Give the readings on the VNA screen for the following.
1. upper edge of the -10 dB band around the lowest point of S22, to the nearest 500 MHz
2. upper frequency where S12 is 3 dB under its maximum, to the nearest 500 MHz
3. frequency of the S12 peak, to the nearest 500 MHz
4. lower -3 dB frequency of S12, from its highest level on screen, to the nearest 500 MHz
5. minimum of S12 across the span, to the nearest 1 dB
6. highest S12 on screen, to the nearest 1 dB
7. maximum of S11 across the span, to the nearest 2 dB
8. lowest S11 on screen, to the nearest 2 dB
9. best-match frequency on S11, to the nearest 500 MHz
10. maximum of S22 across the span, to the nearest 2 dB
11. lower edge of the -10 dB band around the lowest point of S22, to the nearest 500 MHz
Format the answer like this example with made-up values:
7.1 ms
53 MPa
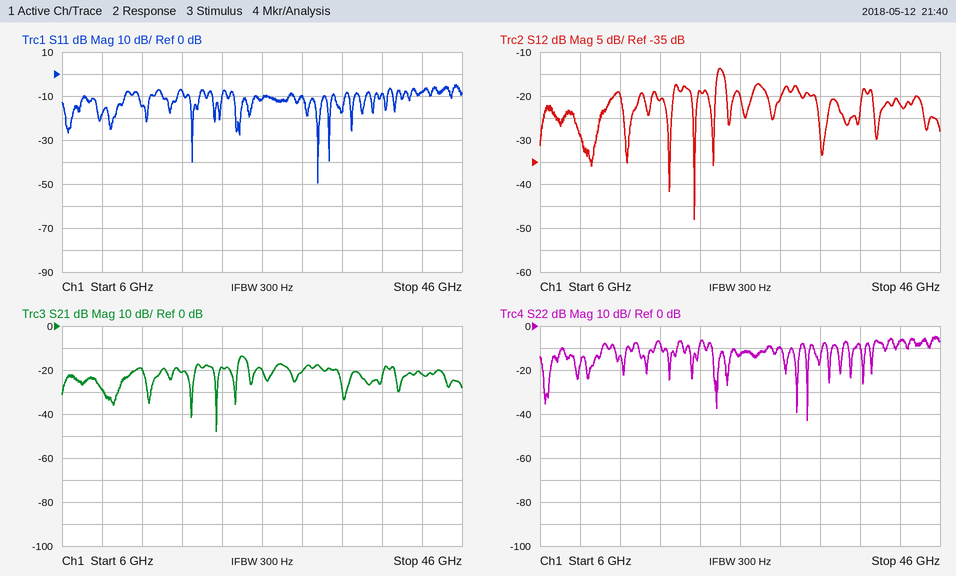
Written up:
33.0 GHz
24.5 GHz
24.0 GHz
23.5 GHz
-48 dB
-14 dB
-4 dB
-50 dB
31.5 GHz
-4 dB
32.5 GHz
